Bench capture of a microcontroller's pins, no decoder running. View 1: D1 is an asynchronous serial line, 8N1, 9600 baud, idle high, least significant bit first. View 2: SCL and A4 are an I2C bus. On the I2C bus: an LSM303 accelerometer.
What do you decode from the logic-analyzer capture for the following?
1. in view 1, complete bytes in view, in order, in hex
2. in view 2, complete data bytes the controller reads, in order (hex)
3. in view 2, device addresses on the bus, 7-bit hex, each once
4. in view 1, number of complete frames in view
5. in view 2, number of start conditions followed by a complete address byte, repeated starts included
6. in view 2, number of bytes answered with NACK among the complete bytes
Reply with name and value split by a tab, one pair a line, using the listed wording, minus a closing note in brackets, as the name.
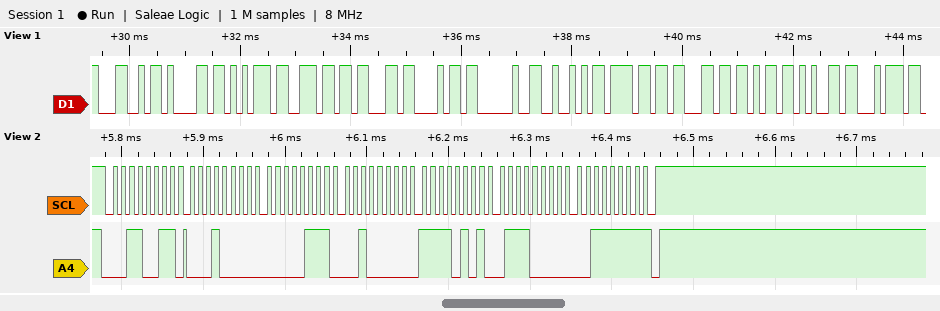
in view 1, complete bytes in view, in order, in hex	4C 61 75 6E 63 68 20 52 6F 63 6B 65 74
in view 2, complete data bytes the controller reads, in order	10 07 20 F5 70 3F
in view 2, device addresses on the bus, 7-bit hex, each once	0x19
in view 1, number of complete frames in view	13
in view 2, number of start conditions followed by a complete address byte, repeated starts included	1
in view 2, number of bytes answered with NACK among the complete bytes	1
